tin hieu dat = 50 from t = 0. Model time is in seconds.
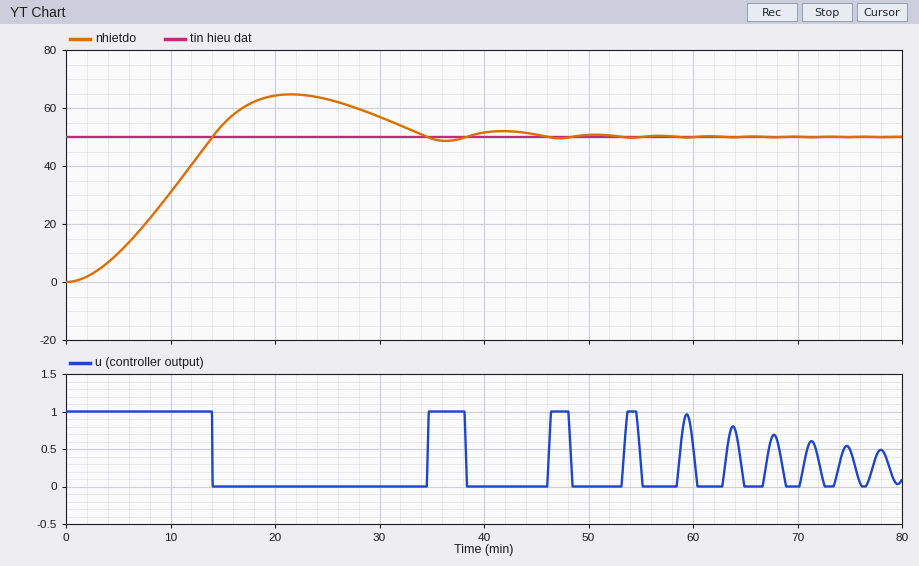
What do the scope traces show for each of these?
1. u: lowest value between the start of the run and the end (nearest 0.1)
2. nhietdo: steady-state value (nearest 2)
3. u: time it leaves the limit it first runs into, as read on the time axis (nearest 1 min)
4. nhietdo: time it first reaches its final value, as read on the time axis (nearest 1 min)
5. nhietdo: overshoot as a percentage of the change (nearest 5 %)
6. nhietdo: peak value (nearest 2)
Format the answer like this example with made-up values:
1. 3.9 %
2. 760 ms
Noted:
1. 0.0
2. 50
3. 14 min
4. 14 min
5. 30 %
6. 64
